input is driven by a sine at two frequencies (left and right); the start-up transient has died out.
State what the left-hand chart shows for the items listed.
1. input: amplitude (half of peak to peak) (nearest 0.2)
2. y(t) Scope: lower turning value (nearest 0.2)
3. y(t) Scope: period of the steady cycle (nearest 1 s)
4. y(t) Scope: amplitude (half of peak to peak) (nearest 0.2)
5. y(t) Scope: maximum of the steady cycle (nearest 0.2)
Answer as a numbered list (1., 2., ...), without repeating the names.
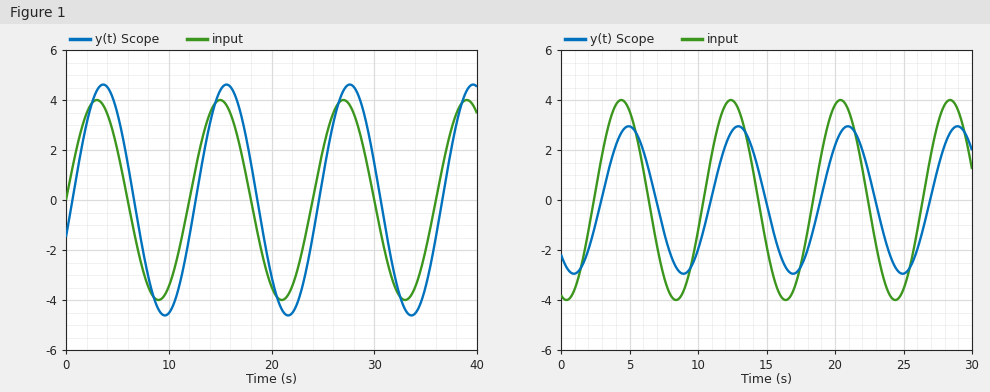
1. 4.0
2. -4.6
3. 12 s
4. 4.6
5. 4.6
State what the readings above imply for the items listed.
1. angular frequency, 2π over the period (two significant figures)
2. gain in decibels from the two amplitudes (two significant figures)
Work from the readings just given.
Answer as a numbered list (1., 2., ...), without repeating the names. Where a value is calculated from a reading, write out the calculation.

1. 2π / 12 = 0.52 rad/s
2. 20 log10(4.6 / 4) = 1.2 dB
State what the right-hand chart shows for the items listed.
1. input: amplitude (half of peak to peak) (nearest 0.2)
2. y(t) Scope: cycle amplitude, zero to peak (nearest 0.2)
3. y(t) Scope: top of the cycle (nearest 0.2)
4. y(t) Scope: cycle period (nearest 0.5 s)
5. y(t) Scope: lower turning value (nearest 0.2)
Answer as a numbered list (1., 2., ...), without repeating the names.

1. 4.0
2. 3.0
3. 3.0
4. 8.0 s
5. -3.0
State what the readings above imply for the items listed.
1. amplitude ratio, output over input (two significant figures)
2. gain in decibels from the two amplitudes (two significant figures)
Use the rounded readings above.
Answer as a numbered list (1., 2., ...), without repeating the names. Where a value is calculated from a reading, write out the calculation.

1. 3 / 4 = 0.75
2. 20 log10(3 / 4) = -2.5 dB
